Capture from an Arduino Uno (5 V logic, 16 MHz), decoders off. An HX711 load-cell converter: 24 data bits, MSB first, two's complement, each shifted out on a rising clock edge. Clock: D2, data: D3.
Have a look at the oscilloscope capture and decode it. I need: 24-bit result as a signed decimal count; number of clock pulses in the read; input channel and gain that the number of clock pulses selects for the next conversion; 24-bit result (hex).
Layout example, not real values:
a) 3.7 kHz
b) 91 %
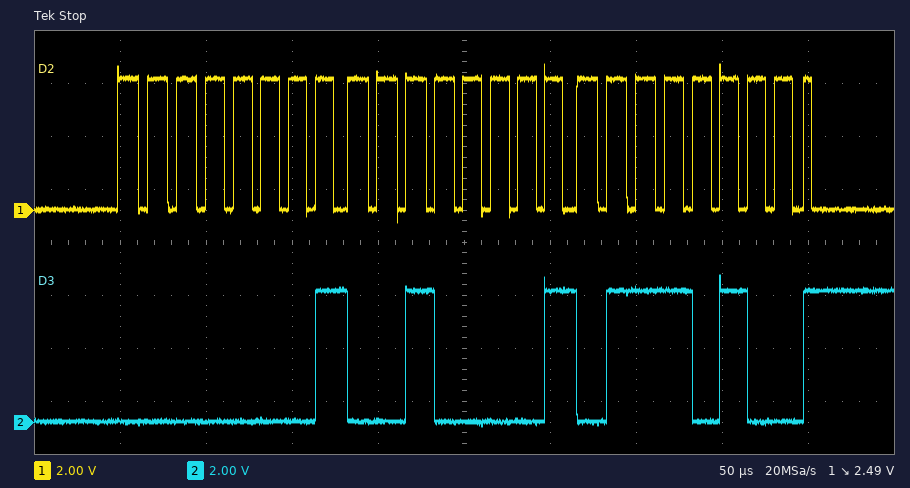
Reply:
a) 74100
b) 25
c) channel A, gain 128
d) 0x012174
